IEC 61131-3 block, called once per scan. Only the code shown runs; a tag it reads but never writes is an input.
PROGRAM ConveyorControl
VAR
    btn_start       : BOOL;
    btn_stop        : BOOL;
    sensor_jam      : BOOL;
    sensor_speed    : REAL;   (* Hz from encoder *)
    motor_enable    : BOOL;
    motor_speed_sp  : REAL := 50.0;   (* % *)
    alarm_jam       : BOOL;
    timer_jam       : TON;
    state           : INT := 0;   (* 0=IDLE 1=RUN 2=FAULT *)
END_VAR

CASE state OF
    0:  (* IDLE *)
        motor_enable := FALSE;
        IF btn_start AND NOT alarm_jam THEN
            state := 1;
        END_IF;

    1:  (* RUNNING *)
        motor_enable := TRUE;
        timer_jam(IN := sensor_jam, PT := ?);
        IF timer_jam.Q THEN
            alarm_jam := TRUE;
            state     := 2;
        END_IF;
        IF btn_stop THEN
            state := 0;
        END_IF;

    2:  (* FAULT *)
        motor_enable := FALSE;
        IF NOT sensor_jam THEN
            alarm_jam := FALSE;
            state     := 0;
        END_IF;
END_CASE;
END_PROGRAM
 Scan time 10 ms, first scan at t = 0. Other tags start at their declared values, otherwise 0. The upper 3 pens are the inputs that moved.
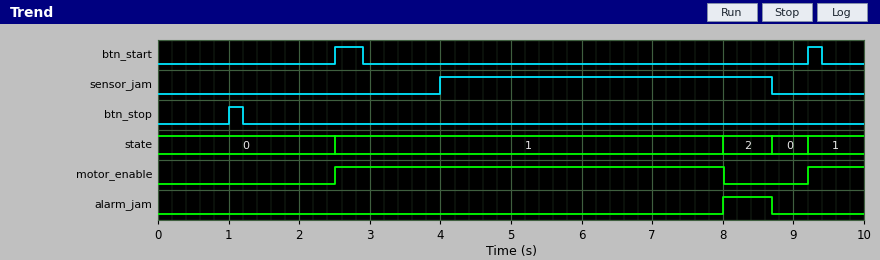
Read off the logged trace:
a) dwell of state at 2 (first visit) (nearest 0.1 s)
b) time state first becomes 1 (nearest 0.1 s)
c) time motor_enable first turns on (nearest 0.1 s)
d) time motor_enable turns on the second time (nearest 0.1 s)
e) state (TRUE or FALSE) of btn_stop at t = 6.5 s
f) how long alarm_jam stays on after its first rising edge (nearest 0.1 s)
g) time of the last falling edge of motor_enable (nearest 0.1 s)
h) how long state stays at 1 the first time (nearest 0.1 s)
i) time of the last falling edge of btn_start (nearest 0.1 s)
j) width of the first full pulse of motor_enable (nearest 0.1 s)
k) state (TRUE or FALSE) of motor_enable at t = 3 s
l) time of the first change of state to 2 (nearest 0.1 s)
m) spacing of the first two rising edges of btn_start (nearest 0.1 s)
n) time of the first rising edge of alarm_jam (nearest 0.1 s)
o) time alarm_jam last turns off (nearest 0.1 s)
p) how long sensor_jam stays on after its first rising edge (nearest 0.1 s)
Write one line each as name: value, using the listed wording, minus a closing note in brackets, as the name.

dwell of state at 2 (first visit): 0.7 s
time state first becomes 1: 2.5 s
time motor_enable first turns on: 2.5 s
time motor_enable turns on the second time: 9.2 s
state (TRUE or FALSE) of btn_stop at t = 6.5 s: FALSE
how long alarm_jam stays on after its first rising edge: 0.7 s
time of the last falling edge of motor_enable: 8.0 s
how long state stays at 1 the first time: 5.5 s
time of the last falling edge of btn_start: 9.4 s
width of the first full pulse of motor_enable: 5.5 s
state (TRUE or FALSE) of motor_enable at t = 3 s: TRUE
time of the first change of state to 2: 8.0 s
spacing of the first two rising edges of btn_start: 6.7 s
time of the first rising edge of alarm_jam: 8.0 s
time alarm_jam last turns off: 8.7 s
how long sensor_jam stays on after its first rising edge: 4.7 s
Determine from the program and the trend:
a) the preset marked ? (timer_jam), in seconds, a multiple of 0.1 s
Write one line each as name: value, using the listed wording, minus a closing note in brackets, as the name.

the preset marked ? (timer_jam), in seconds, a multiple of 0.1 s: 4.0 s
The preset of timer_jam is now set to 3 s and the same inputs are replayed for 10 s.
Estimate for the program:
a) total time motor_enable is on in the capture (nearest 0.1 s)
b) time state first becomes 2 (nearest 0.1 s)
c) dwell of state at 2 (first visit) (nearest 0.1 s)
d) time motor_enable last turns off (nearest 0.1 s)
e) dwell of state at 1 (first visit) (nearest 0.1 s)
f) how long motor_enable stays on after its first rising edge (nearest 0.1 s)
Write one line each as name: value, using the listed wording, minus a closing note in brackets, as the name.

total time motor_enable is on in the capture: 5.3 s
time state first becomes 2: 7.0 s
dwell of state at 2 (first visit): 1.7 s
time motor_enable last turns off: 7.0 s
dwell of state at 1 (first visit): 4.5 s
how long motor_enable stays on after its first rising edge: 4.5 s
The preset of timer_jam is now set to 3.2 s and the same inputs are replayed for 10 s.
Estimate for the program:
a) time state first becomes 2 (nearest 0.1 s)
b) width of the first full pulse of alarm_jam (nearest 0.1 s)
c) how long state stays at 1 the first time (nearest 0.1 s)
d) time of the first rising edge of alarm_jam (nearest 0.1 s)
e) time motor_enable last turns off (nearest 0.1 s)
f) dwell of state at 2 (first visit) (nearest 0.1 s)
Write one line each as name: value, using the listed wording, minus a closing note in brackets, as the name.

time state first becomes 2: 7.2 s
width of the first full pulse of alarm_jam: 1.5 s
how long state stays at 1 the first time: 4.7 s
time of the first rising edge of alarm_jam: 7.2 s
time motor_enable last turns off: 7.2 s
dwell of state at 2 (first visit): 1.5 s
